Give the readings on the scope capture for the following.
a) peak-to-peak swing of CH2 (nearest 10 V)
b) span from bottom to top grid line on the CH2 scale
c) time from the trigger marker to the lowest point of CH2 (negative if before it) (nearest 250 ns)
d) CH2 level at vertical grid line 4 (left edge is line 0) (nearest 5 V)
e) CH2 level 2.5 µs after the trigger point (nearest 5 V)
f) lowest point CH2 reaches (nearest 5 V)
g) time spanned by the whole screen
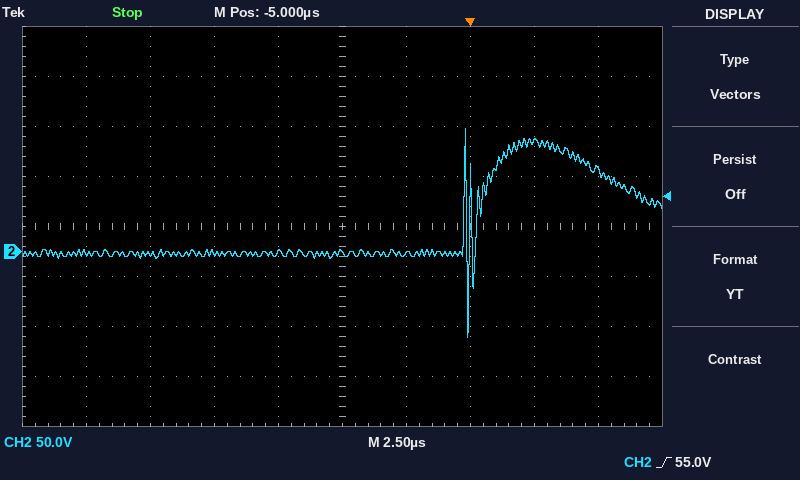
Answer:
210 V
400 V
0.00 µs
0 V
110 V
-85 V
25 µs
